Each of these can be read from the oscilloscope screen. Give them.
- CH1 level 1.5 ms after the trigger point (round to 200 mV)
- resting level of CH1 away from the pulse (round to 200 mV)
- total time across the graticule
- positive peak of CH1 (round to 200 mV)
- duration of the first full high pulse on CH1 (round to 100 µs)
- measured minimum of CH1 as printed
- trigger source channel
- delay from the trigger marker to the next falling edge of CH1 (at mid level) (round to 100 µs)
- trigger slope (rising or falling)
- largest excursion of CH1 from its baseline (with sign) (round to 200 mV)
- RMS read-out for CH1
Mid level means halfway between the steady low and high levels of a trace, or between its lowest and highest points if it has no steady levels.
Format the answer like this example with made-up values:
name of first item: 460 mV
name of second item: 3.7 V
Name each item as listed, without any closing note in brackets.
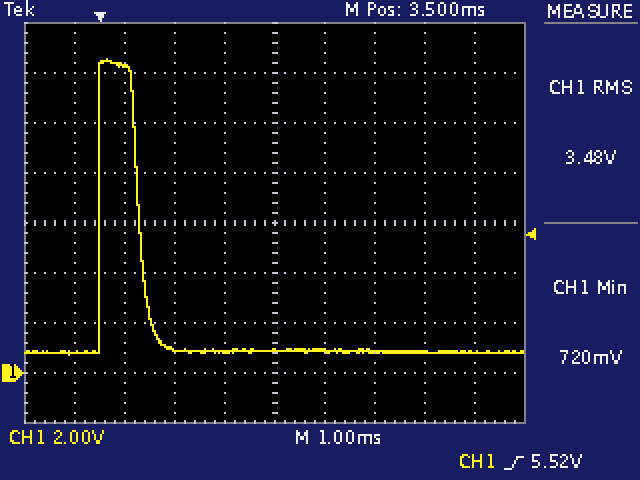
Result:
CH1 level 1.5 ms after the trigger point: 1.0 V
resting level of CH1 away from the pulse: 800 mV
total time across the graticule: 10 ms
positive peak of CH1: 12.6 V
duration of the first full high pulse on CH1: 800 µs
measured minimum of CH1 as printed: 720 mV
trigger source channel: CH1
delay from the trigger marker to the next falling edge of CH1 (at mid level): 800 µs
trigger slope: rising
largest excursion of CH1 from its baseline (with sign): +11.8 V
RMS read-out for CH1: 3.48 V
